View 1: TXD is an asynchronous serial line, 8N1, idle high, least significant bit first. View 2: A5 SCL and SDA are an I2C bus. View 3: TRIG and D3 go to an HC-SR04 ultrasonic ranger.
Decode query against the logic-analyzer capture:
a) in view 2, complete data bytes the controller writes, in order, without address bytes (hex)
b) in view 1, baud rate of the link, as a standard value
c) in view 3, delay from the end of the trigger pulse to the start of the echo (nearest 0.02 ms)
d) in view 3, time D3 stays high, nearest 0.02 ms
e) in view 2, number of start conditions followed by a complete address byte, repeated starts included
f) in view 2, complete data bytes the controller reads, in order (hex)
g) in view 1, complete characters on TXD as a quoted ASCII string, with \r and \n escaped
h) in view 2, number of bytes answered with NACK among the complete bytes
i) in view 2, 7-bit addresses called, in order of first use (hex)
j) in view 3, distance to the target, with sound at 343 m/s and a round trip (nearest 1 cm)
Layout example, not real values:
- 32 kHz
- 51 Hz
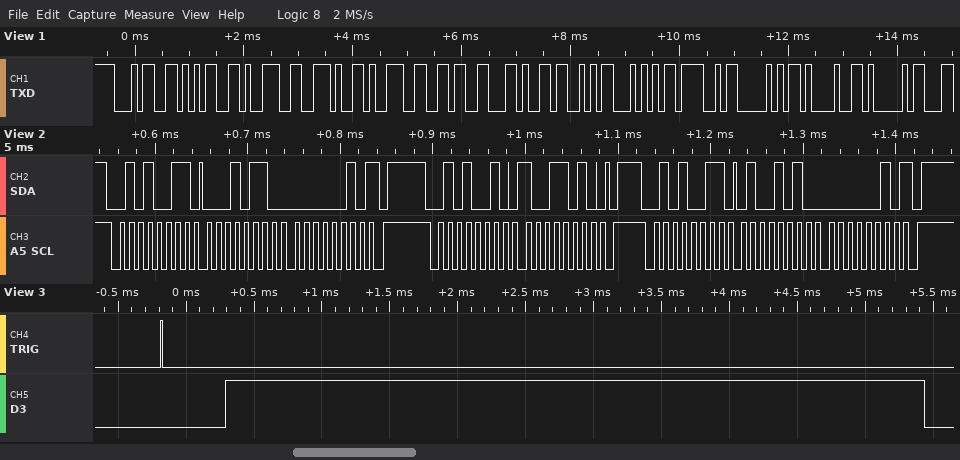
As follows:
- 9A
- 9600 baud
- 0.46 ms
- 5.14 ms
- 3
- 16 02 4A 02
- "459.96,STOP!A"
- 2
- 0x29
- 88 cm
